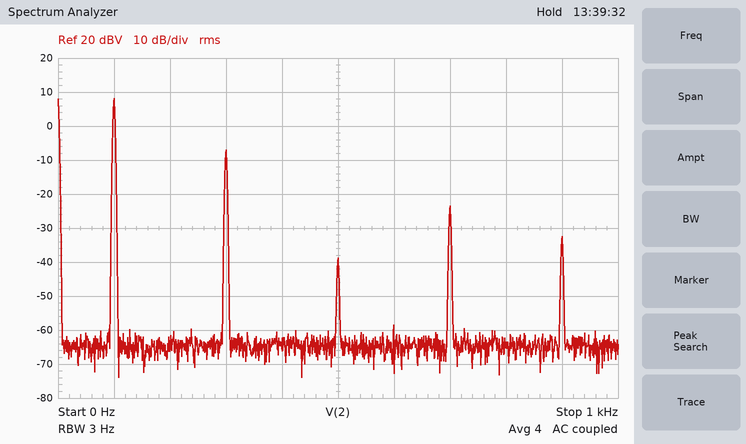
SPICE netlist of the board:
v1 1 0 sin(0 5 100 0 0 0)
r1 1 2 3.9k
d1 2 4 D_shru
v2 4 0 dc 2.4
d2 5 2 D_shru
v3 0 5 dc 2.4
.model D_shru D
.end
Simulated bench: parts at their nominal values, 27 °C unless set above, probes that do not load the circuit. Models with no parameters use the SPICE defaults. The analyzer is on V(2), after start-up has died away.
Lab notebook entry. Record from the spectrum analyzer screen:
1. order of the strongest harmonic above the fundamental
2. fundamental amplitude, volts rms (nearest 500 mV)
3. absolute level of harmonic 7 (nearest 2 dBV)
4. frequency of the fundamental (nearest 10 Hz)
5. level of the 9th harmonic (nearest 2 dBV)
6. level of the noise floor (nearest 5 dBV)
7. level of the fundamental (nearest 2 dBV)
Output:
3
2.5 V
-24 dBV
100 Hz
-32 dBV
-65 dBV
8 dBV
